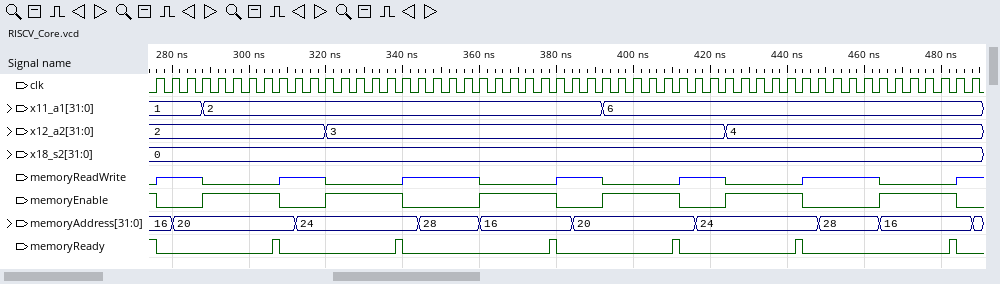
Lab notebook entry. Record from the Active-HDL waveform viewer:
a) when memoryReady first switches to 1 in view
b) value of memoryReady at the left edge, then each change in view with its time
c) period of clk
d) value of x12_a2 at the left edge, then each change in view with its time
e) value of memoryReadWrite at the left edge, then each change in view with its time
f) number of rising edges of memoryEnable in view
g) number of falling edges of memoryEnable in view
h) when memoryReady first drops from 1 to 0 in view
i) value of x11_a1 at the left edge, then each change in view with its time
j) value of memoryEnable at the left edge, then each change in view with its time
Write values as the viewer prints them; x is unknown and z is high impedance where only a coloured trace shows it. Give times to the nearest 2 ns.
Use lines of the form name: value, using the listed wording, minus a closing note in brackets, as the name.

when memoryReady first switches to 1 in view: 306 ns
value of memoryReady at the left edge, then each change in view with its time: 1, 0 at 276 ns, 1 at 306 ns, 0 at 308 ns, 1 at 338 ns, 0 at 340 ns, 1 at 378 ns, 0 at 380 ns, 1 at 410 ns, 0 at 412 ns, 1 at 442 ns, 0 at 444 ns, 1 at 482 ns, 0 at 484 ns
period of clk: 4 ns
value of x12_a2 at the left edge, then each change in view with its time: 2, 3 at 320 ns, 4 at 424 ns
value of memoryReadWrite at the left edge, then each change in view with its time: 0, z at 276 ns, 0 at 288 ns, z at 308 ns, 0 at 320 ns, z at 340 ns, 0 at 360 ns, z at 380 ns, 0 at 392 ns, z at 412 ns, 0 at 424 ns, z at 444 ns, 0 at 464 ns, z at 484 ns
number of rising edges of memoryEnable in view: 6
number of falling edges of memoryEnable in view: 7
when memoryReady first drops from 1 to 0 in view: 276 ns
value of x11_a1 at the left edge, then each change in view with its time: 1, 2 at 288 ns, 6 at 392 ns
value of memoryEnable at the left edge, then each change in view with its time: 1, 0 at 276 ns, 1 at 288 ns, 0 at 308 ns, 1 at 320 ns, 0 at 340 ns, 1 at 360 ns, 0 at 380 ns, 1 at 392 ns, 0 at 412 ns, 1 at 424 ns, 0 at 444 ns, 1 at 464 ns, 0 at 484 ns
